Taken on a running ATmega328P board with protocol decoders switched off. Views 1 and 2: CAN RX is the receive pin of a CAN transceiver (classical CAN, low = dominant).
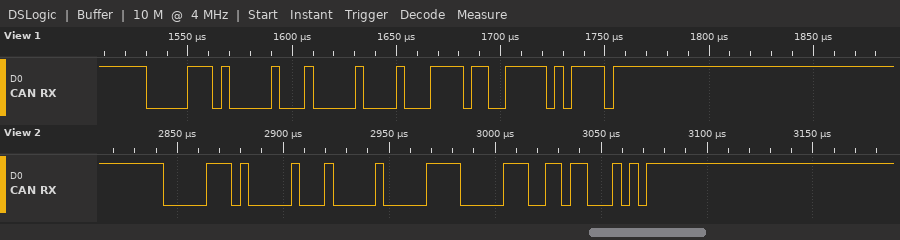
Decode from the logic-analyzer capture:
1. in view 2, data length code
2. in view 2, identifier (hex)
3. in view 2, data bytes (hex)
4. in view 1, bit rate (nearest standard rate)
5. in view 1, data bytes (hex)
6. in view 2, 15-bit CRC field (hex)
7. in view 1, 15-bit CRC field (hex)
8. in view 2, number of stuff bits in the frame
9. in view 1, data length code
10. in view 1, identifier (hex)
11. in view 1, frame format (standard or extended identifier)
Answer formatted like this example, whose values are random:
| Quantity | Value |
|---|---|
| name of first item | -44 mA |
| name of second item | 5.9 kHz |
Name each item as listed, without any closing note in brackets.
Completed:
| Quantity | Value |
|---|---|
| in view 2, data length code | 2 |
| in view 2, identifier | 0x068 |
| in view 2, data bytes | 00 70 |
| in view 1, bit rate | 250 kbit/s |
| in view 1, data bytes | 00 8F |
| in view 2, 15-bit CRC field | 0x3362 |
| in view 1, 15-bit CRC field | 0x33F7 |
| in view 2, number of stuff bits in the frame | 5 |
| in view 1, data length code | 2 |
| in view 1, identifier | 0x068 |
| in view 1, frame format | standard |
